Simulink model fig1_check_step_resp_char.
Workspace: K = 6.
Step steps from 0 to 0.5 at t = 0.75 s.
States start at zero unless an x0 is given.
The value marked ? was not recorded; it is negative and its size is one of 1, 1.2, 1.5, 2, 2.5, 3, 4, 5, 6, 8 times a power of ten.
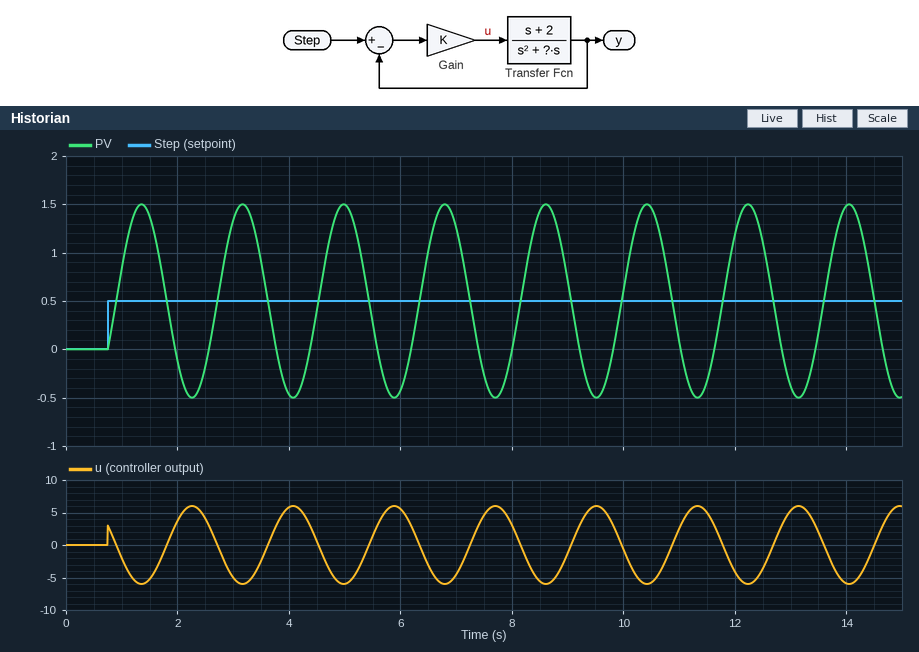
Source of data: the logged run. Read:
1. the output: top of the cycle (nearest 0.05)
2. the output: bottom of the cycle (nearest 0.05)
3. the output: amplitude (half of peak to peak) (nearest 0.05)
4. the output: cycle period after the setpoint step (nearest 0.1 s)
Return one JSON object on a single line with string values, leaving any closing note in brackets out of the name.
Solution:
{"the output: top of the cycle": "1.50", "the output: bottom of the cycle": "-0.50", "the output: amplitude (half of peak to peak)": "1.00", "the output: cycle period after the setpoint step": "1.8 s"}
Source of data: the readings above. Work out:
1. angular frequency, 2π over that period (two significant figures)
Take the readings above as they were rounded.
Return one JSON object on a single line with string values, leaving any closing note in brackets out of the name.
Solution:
{"angular frequency, 2π over that period": "3.5 rad/s"}
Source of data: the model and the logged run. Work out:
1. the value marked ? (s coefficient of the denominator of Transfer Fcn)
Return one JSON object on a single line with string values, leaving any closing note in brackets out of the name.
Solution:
{"the value marked ?": "-6"}
